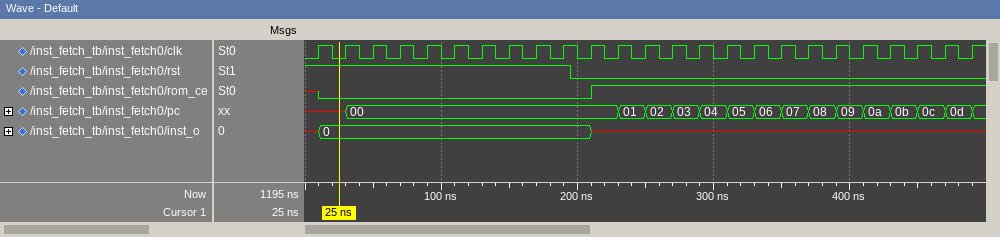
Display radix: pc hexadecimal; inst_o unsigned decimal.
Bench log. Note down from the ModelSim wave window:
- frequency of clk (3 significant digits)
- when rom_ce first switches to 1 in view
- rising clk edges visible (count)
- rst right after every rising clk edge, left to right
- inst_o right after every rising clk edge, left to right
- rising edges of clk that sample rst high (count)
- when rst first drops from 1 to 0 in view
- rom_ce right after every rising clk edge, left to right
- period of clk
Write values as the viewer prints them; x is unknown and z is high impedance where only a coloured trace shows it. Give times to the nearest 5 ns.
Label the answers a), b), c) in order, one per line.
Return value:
a) 50.0 MHz
b) 210 ns
c) 25
d) 1 1 1 1 1 1 1 1 1 1 0 0 0 0 0 0 0 0 0 0 0 0 0 0 0
e) 0, 0, 0, 0, 0, 0, 0, 0, 0, 0, x, x, x, x, x, x, x, x, x, x, x, x, x, x, x
f) 10
g) 195 ns
h) 0 0 0 0 0 0 0 0 0 0 1 1 1 1 1 1 1 1 1 1 1 1 1 1 1
i) 20 ns
